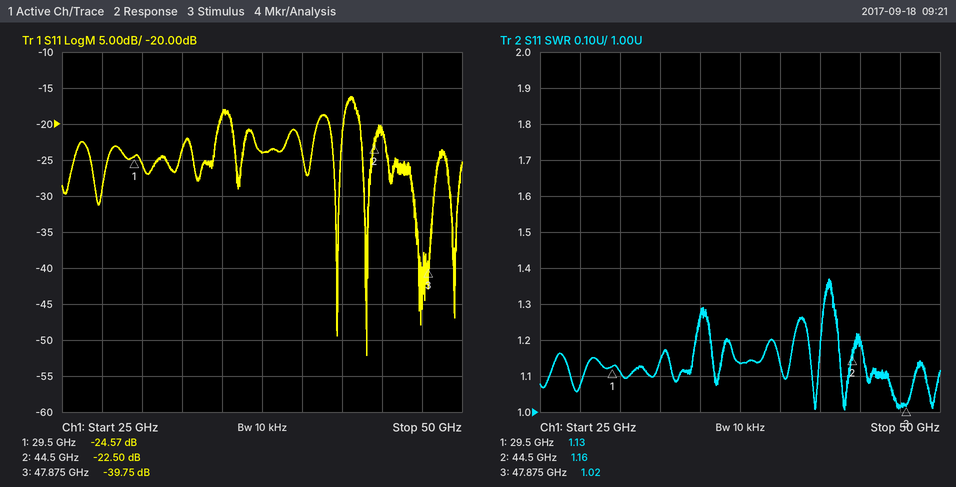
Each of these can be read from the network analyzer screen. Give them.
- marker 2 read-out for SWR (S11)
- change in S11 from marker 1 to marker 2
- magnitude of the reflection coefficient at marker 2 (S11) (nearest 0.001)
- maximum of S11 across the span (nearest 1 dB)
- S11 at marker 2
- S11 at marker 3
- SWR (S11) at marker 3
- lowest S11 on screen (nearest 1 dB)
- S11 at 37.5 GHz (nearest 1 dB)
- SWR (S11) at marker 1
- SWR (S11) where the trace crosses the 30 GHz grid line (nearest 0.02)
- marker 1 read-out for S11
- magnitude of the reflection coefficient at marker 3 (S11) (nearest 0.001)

1.16
2.07 dB
0.075
-16 dB
-22.50 dB
-39.75 dB
1.02
-52 dB
-24 dB
1.13
1.12
-24.57 dB
0.010
